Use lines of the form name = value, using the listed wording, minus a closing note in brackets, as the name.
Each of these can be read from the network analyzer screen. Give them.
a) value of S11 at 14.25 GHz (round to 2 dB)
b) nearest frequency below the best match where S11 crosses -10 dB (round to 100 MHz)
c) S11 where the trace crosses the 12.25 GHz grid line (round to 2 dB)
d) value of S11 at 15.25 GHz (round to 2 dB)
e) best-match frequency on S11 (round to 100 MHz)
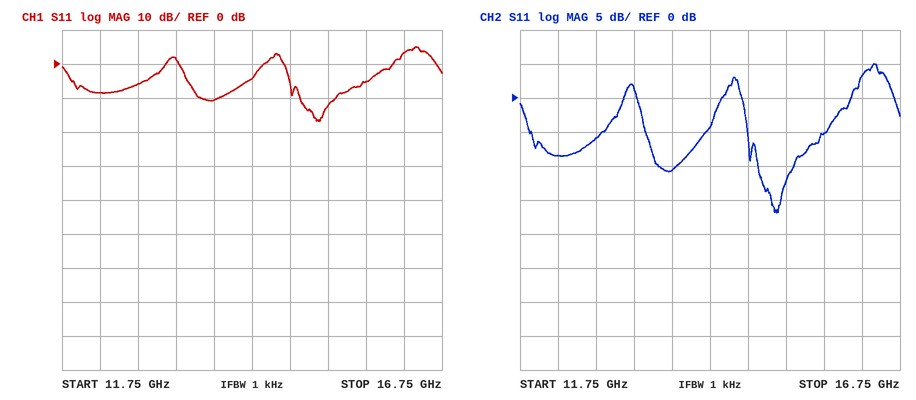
value of S11 at 14.25 GHz = -4 dB
nearest frequency below the best match where S11 crosses -10 dB = 14.9 GHz
S11 where the trace crosses the 12.25 GHz grid line = -8 dB
value of S11 at 15.25 GHz = -12 dB
best-match frequency on S11 = 15.1 GHz
